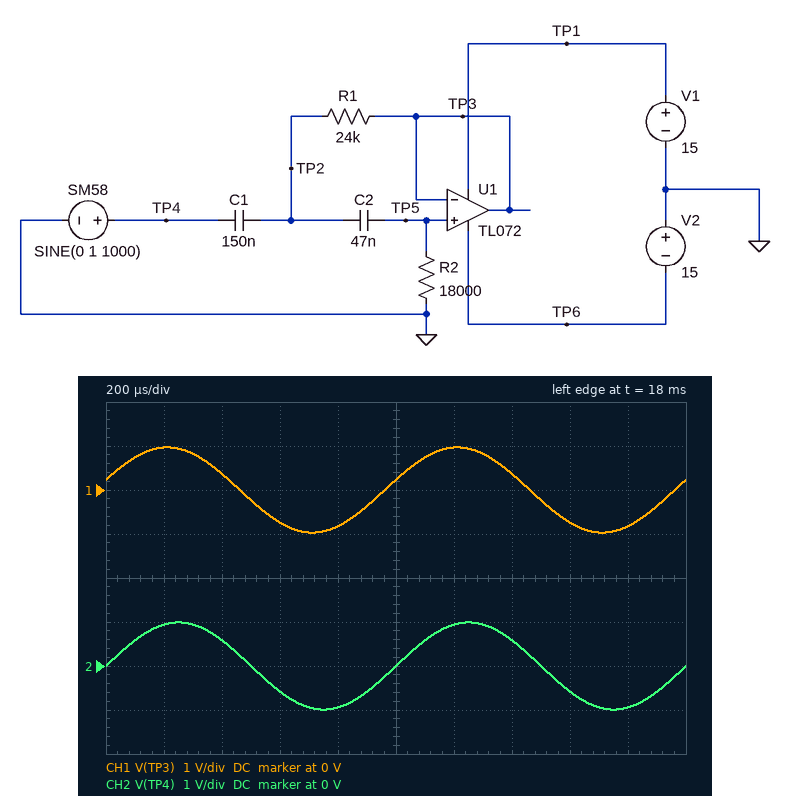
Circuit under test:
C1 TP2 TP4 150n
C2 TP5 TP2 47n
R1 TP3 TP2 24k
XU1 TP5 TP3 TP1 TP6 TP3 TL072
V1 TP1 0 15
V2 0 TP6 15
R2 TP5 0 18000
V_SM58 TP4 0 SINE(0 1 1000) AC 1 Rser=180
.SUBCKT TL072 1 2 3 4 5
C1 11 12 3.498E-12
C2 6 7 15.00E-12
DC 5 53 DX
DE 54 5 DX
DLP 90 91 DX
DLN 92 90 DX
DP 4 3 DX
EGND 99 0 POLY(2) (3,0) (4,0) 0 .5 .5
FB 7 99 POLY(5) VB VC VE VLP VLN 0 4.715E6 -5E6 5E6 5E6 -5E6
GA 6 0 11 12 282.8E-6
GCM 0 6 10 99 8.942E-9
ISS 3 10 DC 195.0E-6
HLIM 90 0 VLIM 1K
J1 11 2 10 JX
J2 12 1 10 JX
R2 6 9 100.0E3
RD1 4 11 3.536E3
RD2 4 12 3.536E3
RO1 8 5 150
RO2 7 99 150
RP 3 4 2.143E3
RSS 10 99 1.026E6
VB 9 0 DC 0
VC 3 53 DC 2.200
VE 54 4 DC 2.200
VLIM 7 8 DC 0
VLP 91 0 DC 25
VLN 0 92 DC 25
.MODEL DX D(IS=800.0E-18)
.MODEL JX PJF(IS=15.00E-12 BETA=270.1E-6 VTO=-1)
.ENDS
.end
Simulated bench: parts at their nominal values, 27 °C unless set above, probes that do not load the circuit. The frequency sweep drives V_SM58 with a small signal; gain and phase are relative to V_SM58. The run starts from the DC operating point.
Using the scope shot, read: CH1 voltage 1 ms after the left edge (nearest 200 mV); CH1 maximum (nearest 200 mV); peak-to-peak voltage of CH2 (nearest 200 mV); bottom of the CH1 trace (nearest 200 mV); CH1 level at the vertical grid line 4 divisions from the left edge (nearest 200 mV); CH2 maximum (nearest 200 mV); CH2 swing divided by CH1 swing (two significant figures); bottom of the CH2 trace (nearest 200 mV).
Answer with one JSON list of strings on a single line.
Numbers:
["200 mV", "1.0 V", "2.0 V", "-1.0 V", "-800 mV", "1.0 V", "1.0", "-1.0 V"]
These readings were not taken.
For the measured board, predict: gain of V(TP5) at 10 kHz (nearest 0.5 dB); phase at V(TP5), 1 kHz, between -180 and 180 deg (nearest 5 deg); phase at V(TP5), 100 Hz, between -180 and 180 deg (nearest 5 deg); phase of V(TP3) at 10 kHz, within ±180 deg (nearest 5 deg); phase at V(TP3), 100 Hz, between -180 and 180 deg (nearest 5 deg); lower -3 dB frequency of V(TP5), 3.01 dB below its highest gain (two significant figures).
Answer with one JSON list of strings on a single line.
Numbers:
["0 dB", "15 deg", "85 deg", "0 deg", "85 deg", "210 Hz"]
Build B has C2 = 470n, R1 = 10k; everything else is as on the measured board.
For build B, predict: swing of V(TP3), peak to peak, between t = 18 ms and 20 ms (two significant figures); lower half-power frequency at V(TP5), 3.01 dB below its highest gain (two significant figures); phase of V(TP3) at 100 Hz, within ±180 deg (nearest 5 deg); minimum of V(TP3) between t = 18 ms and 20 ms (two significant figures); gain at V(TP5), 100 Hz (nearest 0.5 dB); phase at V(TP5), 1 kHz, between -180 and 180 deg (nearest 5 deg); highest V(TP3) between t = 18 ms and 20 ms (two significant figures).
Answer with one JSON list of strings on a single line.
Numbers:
["2.0 V", "57 Hz", "45 deg", "-990 mV", "-1.0 dB", "5 deg", "990 mV"]
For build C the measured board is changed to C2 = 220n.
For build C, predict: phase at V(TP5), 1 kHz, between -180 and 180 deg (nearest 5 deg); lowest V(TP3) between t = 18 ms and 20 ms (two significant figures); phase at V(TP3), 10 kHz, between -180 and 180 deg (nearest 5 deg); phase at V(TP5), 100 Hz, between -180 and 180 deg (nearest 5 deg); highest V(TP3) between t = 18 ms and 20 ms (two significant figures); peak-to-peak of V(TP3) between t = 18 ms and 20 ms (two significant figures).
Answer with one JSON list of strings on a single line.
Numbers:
["5 deg", "-990 mV", "0 deg", "50 deg", "990 mV", "2.0 V"]
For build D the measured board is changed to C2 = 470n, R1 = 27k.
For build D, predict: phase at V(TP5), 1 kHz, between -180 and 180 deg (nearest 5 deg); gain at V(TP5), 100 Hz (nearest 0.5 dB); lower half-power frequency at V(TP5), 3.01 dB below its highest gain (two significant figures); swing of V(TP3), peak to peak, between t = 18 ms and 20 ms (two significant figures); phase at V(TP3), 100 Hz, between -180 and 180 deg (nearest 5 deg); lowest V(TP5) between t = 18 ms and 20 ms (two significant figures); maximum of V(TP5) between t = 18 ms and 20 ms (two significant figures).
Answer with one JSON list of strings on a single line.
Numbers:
["5 deg", "-1.5 dB", "68 Hz", "2.0 V", "40 deg", "-990 mV", "990 mV"]
